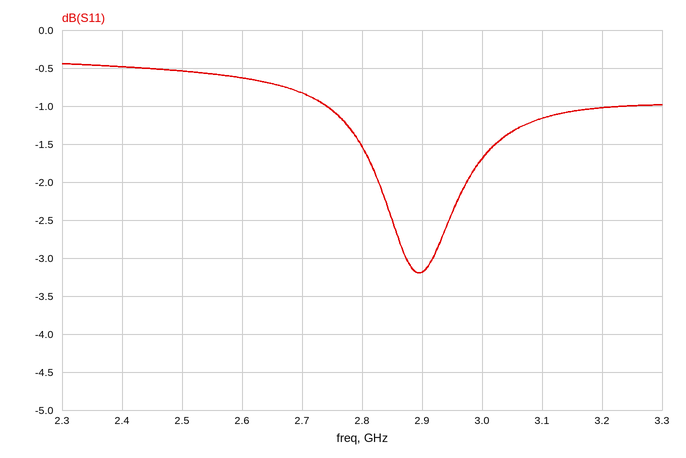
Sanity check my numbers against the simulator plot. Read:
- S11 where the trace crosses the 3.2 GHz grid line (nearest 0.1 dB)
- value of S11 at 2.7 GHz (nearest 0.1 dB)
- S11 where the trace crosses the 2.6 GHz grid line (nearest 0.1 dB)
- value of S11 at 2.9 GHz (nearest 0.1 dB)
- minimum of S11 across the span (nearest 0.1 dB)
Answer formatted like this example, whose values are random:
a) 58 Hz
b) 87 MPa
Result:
a) -1.0 dB
b) -0.8 dB
c) -0.6 dB
d) -3.2 dB
e) -3.2 dB
